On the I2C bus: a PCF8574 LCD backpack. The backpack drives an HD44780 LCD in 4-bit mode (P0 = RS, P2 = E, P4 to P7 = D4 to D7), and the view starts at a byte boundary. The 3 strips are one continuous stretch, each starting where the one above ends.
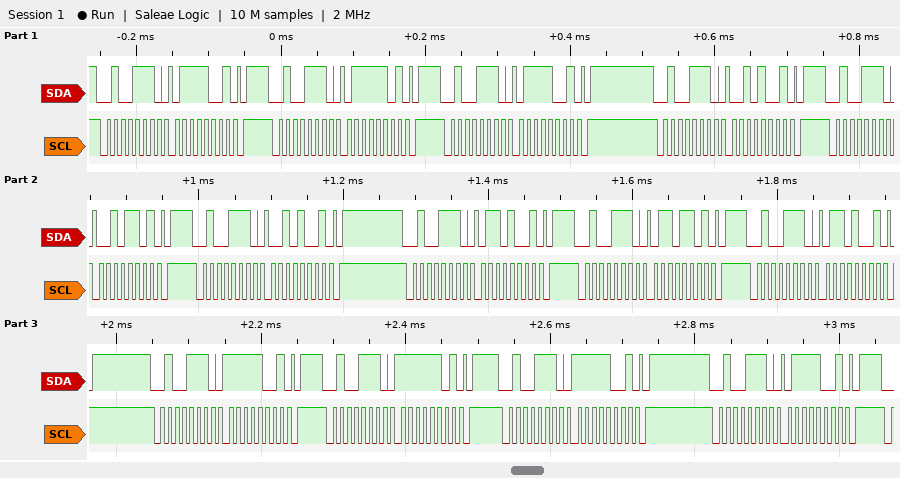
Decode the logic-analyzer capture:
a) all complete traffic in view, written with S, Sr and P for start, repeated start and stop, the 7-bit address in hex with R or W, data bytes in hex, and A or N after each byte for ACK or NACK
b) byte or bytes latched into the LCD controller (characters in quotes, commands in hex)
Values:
S 27W A 79 A P S 27W A 7D A P S 27W A 79 A P S 27W A 29 A P S 27W A 2D A P S 27W A 29 A P S 27W A 69 A P S 27W A 6D A P S 27W A 69 A P S 27W A F9 A P S 27W A FD A P S 27W A F9 A P S 27W A 79 A P
'r' 'o'
